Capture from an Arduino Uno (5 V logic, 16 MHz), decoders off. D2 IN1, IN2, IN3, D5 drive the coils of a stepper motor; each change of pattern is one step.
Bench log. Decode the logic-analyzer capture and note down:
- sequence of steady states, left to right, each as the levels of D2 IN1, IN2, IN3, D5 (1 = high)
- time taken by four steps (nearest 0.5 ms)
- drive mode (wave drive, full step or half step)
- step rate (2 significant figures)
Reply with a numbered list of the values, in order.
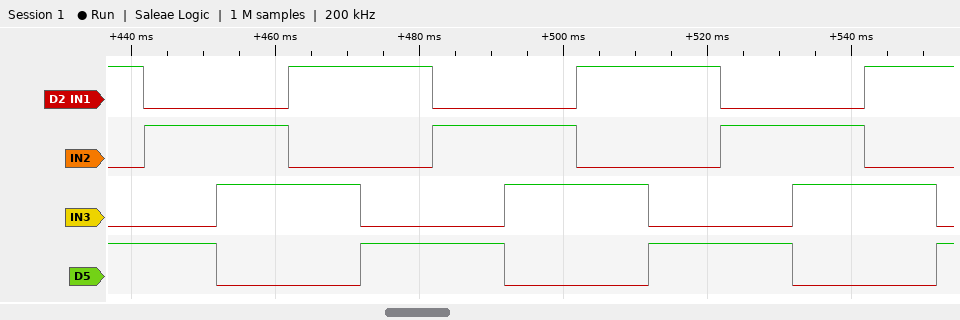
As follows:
1. 1001 0101 0110 1010 1001 0101 0110 1010 1001 0101 0110 1010 1001
2. 40.0 ms
3. full step
4. 100 steps/s
